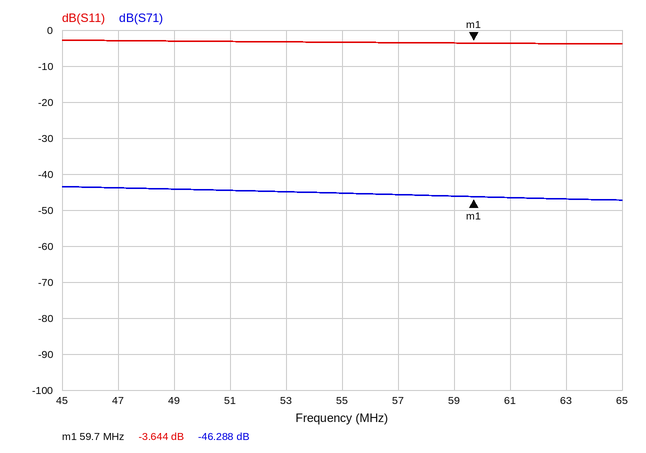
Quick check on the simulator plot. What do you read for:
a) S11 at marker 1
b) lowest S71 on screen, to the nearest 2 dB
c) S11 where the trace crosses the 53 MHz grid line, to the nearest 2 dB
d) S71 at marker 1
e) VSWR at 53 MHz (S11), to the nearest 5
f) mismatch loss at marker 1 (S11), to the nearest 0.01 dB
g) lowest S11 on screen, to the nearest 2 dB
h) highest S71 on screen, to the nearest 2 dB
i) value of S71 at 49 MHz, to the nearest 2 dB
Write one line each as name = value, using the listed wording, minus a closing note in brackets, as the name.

S11 at marker 1 = -3.644 dB
lowest S71 on screen, to the nearest 2 dB = -48 dB
S11 where the trace crosses the 53 MHz grid line, to the nearest 2 dB = -4 dB
S71 at marker 1 = -46.288 dB
VSWR at 53 MHz (S11), to the nearest 5 = 5
mismatch loss at marker 1 (S11), to the nearest 0.01 dB = 2.46 dB
lowest S11 on screen, to the nearest 2 dB = -4 dB
highest S71 on screen, to the nearest 2 dB = -44 dB
value of S71 at 49 MHz, to the nearest 2 dB = -44 dB
